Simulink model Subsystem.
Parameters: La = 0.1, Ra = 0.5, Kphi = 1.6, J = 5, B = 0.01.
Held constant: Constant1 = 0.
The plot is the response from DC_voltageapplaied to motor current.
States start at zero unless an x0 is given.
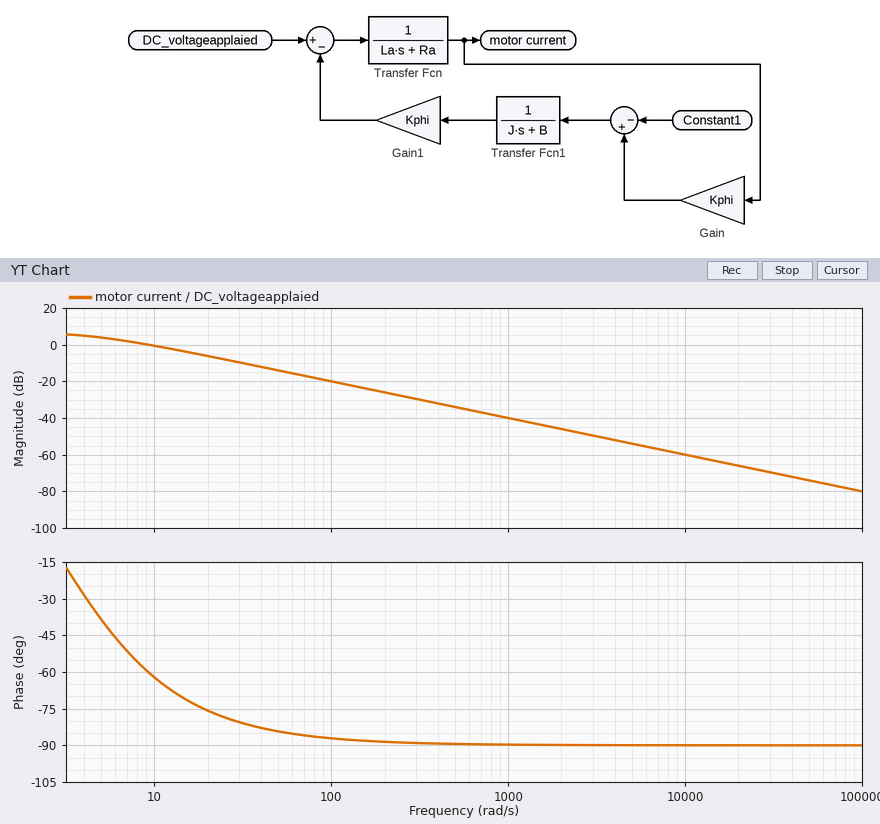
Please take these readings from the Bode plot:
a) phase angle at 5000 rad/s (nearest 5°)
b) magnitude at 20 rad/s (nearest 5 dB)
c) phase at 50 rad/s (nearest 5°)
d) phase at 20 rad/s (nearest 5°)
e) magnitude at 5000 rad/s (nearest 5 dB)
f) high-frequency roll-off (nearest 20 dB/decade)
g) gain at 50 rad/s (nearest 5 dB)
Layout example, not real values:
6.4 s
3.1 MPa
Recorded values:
-90°
-5 dB
-85°
-75°
-55 dB
-20 dB/decade
-15 dB
